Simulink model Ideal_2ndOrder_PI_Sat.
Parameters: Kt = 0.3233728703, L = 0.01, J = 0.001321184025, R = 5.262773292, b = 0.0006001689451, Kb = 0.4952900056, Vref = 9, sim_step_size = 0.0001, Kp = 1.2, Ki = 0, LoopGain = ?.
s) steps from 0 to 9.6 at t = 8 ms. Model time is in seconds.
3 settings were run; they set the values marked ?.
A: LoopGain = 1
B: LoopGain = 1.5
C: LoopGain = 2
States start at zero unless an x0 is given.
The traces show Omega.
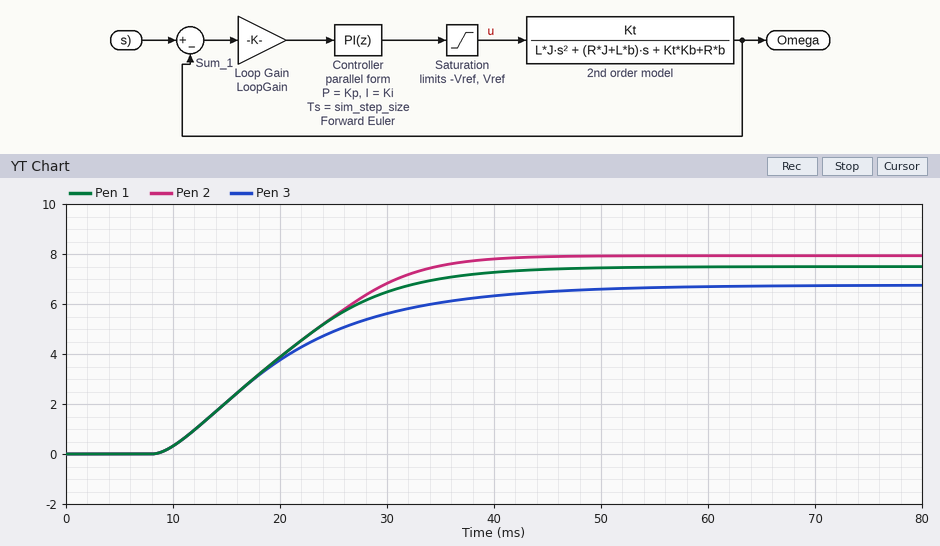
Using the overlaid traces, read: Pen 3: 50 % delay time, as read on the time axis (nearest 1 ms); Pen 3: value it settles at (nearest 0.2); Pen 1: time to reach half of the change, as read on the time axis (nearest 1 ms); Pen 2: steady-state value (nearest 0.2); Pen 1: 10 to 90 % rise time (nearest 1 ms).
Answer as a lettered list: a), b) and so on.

a) 19 ms
b) 6.8
c) 20 ms
d) 8.0
e) 21 ms
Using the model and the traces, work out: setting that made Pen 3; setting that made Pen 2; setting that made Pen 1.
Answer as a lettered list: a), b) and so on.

a) A
b) C
c) B
